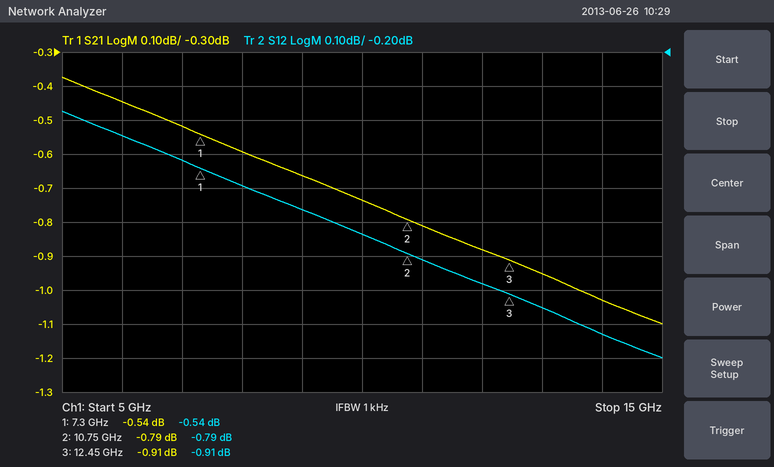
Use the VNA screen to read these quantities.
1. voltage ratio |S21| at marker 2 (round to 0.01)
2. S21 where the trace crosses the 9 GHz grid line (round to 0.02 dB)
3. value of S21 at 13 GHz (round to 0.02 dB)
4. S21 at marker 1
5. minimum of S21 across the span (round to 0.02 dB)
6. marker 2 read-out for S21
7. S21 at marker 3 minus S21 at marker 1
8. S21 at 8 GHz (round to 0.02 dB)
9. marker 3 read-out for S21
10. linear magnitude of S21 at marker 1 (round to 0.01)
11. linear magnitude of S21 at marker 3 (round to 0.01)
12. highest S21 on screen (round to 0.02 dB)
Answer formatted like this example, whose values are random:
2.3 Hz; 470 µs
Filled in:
0.91; -0.66 dB; -0.96 dB; -0.54 dB; -1.10 dB; -0.79 dB; -0.37 dB; -0.60 dB; -0.91 dB; 0.94; 0.90; -0.38 dB
